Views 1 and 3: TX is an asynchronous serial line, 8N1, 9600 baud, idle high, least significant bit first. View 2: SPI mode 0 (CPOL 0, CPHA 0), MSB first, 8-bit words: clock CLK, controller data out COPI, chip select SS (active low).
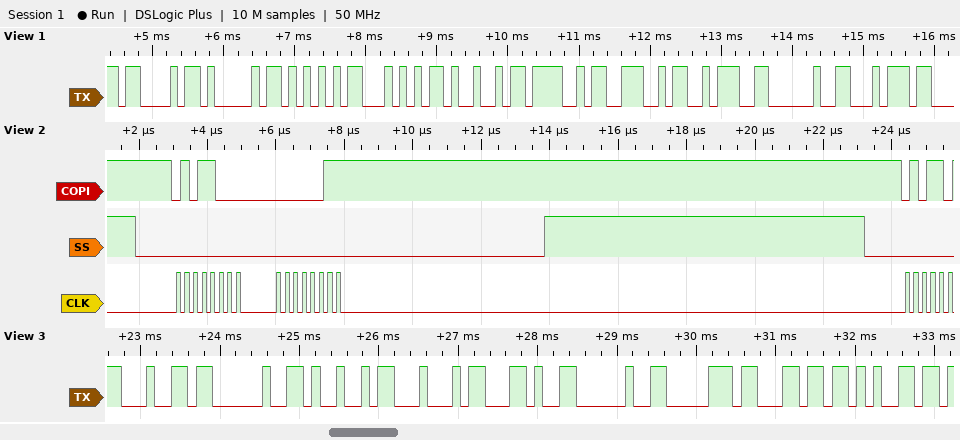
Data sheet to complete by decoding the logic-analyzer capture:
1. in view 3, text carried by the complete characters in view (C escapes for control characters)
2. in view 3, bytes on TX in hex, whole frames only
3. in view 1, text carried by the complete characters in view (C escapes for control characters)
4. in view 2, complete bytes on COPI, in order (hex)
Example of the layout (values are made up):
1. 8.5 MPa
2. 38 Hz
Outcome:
1. "d ID, ple"
2. 64 20 49 44 2C 20 70 6C 65
3. "CAUTION: t"
4. 58 03
